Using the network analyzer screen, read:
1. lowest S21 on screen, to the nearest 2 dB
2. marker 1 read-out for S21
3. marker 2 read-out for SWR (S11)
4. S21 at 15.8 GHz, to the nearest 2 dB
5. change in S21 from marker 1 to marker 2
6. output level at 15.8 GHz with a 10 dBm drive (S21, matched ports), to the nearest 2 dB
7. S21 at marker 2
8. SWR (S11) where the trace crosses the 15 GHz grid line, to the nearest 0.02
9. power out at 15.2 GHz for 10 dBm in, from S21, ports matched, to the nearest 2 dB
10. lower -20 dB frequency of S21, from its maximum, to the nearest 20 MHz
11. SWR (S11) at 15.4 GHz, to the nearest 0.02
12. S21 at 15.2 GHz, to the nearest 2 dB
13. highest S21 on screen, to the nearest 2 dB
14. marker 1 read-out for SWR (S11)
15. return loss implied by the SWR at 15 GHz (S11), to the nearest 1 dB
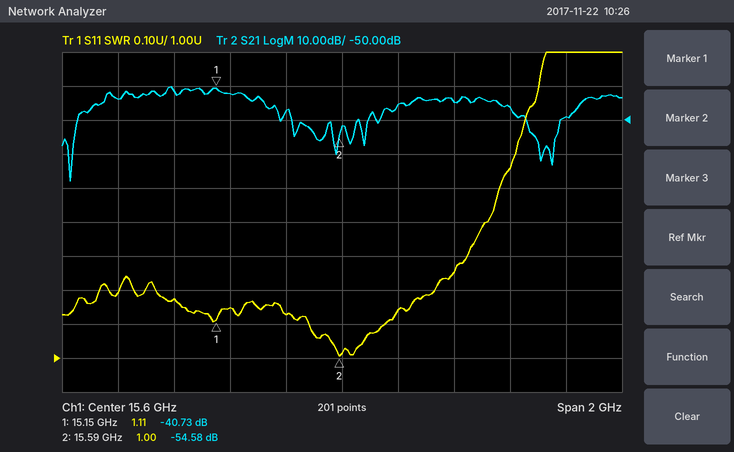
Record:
-68 dB
-40.73 dB
1.00
-46 dB
-13.85 dB
-36 dBm
-54.58 dB
1.18
-32 dBm
14.64 GHz
1.12
-42 dB
-40 dB
1.11
22 dB
